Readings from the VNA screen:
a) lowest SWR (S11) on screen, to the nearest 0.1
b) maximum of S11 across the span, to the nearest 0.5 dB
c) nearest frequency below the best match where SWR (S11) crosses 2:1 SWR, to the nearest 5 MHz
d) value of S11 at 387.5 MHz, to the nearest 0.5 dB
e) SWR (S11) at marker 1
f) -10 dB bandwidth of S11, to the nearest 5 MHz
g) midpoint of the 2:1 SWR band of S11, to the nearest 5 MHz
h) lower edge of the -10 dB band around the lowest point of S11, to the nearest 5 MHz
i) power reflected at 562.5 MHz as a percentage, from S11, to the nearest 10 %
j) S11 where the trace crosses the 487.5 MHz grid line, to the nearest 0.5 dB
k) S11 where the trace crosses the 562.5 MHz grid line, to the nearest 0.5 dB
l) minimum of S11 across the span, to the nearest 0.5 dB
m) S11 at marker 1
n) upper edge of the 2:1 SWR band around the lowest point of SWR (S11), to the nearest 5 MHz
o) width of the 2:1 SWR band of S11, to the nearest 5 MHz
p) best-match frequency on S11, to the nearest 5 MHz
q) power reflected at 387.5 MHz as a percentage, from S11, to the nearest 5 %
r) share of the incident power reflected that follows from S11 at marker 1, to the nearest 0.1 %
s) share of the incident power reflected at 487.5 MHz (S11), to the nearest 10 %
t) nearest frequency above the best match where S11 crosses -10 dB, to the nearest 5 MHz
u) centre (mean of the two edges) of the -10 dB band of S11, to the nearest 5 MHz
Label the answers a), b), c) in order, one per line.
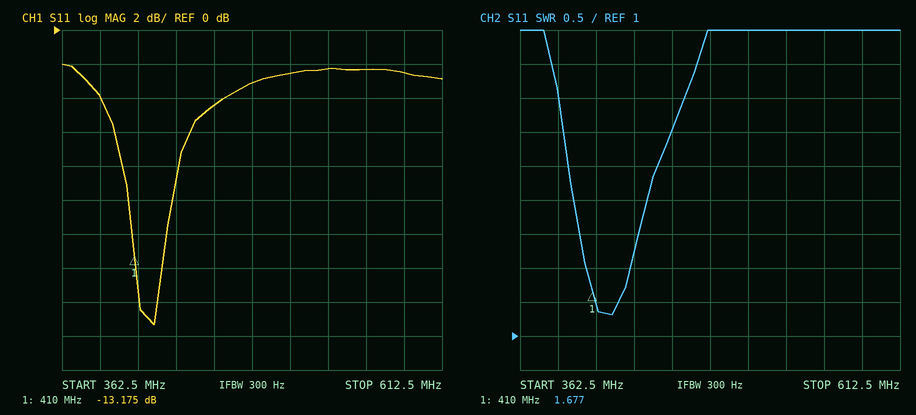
a) 1.3
b) -2.0 dB
c) 405 MHz
d) -4.0 dB
e) 1.677
f) 30 MHz
g) 420 MHz
h) 405 MHz
i) 60 %
j) -3.0 dB
k) -2.5 dB
l) -17.5 dB
m) -13.175 dB
n) 435 MHz
o) 30 MHz
p) 425 MHz
q) 40 %
r) 4.8 %
s) 50 %
t) 435 MHz
u) 420 MHz
